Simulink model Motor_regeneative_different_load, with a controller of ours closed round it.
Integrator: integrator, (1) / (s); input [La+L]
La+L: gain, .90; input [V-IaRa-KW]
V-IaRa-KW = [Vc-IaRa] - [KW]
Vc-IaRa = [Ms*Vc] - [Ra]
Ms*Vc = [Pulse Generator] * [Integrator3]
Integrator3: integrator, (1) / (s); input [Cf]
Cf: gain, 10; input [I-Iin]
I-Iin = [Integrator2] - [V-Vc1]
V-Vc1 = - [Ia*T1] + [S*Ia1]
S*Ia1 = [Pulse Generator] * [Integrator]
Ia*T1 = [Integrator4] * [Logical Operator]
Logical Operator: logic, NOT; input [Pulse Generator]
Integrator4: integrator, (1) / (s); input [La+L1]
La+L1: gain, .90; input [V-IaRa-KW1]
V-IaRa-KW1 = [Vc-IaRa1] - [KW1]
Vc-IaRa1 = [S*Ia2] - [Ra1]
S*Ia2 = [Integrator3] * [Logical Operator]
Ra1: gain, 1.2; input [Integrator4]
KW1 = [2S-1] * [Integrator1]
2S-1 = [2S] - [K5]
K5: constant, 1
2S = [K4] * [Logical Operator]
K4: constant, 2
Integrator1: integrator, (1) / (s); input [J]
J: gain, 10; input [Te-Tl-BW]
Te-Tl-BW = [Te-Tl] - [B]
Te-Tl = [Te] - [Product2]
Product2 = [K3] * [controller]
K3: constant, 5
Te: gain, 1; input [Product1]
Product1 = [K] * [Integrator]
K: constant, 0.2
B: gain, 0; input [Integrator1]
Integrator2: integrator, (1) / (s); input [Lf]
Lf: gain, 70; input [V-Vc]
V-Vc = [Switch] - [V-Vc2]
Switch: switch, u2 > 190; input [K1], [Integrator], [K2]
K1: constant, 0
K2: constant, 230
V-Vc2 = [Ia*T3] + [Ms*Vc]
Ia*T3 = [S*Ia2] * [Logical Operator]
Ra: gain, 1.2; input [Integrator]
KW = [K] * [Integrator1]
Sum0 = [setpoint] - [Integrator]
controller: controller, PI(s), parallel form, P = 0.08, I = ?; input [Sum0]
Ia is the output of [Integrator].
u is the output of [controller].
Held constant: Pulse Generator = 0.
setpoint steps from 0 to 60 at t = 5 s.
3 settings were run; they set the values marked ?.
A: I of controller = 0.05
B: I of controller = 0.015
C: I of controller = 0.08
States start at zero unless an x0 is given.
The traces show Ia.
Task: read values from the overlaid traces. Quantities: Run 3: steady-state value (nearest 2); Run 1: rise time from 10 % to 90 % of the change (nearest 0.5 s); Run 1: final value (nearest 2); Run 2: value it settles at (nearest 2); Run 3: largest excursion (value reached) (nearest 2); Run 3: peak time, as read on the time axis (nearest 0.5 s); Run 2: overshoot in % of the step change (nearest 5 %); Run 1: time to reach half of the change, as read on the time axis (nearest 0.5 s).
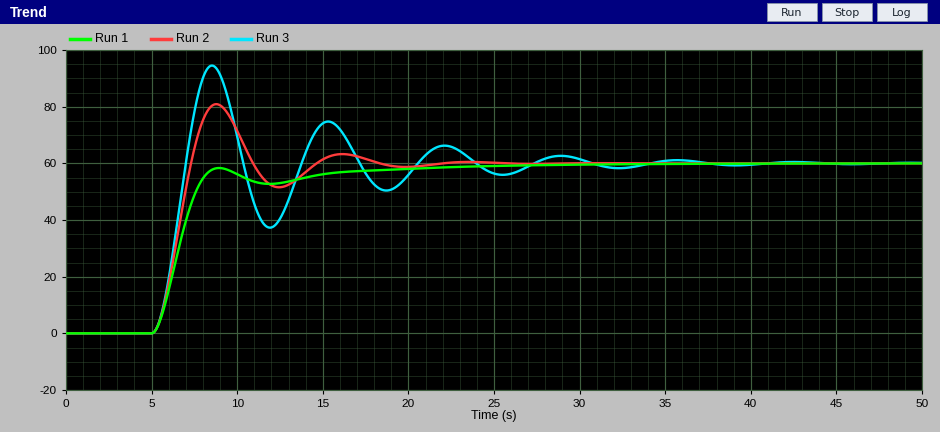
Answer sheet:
60
2.5 s
60
60
94
8.5 s
35 %
6.5 s
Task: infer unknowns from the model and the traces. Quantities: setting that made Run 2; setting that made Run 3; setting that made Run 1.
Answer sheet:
A
C
B
